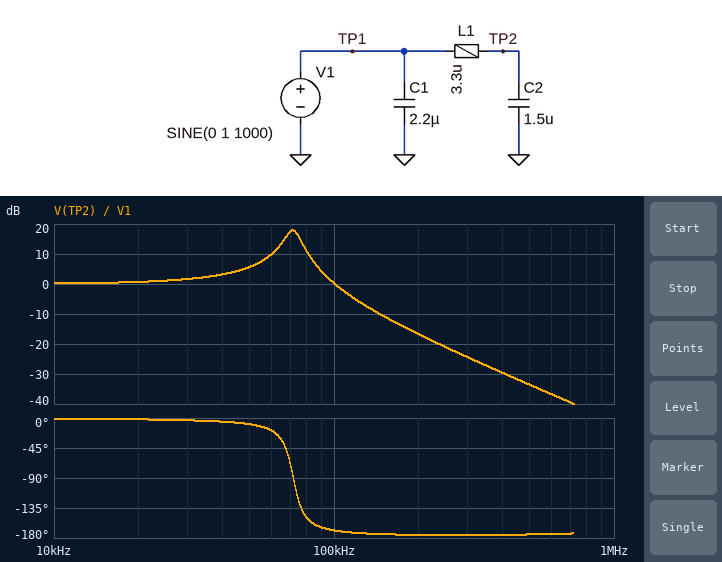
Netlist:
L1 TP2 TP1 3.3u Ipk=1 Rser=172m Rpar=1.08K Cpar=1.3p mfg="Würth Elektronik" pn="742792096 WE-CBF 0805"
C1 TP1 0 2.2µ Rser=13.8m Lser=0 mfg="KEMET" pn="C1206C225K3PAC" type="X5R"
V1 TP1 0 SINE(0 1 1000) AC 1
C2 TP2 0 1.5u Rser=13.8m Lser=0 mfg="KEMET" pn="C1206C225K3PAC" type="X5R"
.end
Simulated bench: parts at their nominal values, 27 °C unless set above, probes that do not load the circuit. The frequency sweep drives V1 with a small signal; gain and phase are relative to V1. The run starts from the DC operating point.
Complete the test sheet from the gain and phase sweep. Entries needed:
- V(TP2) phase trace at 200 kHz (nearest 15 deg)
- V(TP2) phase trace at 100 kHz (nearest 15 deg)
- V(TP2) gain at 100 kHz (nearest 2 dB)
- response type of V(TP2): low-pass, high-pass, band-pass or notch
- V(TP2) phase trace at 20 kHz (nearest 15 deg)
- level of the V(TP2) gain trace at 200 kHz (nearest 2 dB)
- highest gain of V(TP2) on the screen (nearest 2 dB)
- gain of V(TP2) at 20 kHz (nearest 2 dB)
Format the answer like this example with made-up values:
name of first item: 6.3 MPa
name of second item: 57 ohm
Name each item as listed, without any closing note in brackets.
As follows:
V(TP2) phase trace at 200 kHz: -180 deg
V(TP2) phase trace at 100 kHz: -165 deg
V(TP2) gain at 100 kHz: 0 dB
response type of V(TP2): low-pass, high-pass, band-pass or notch: low-pass
V(TP2) phase trace at 20 kHz: 0 deg
level of the V(TP2) gain trace at 200 kHz: -16 dB
highest gain of V(TP2) on the screen: 18 dB
gain of V(TP2) at 20 kHz: 0 dB
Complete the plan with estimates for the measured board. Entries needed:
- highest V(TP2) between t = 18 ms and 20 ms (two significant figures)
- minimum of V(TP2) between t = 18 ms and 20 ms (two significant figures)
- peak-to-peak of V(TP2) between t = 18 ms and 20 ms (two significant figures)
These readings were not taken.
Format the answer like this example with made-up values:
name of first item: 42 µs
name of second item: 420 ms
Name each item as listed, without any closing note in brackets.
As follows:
highest V(TP2) between t = 18 ms and 20 ms: 1.0 V
minimum of V(TP2) between t = 18 ms and 20 ms: -1.0 V
peak-to-peak of V(TP2) between t = 18 ms and 20 ms: 2.0 V
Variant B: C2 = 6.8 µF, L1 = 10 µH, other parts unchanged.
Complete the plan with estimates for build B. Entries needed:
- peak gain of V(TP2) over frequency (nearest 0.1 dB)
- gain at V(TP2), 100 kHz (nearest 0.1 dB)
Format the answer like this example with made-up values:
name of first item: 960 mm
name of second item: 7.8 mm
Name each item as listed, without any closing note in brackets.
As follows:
peak gain of V(TP2) over frequency: 16.3 dB
gain at V(TP2), 100 kHz: -28.2 dB
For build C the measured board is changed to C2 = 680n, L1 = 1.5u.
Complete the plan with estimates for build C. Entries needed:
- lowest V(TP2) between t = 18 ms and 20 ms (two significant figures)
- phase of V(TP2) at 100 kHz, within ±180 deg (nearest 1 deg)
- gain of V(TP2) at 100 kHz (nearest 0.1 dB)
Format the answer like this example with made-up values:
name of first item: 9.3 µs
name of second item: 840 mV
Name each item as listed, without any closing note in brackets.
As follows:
lowest V(TP2) between t = 18 ms and 20 ms: -1.0 V
phase of V(TP2) at 100 kHz, within ±180 deg: -7 deg
gain of V(TP2) at 100 kHz: 4.4 dB
